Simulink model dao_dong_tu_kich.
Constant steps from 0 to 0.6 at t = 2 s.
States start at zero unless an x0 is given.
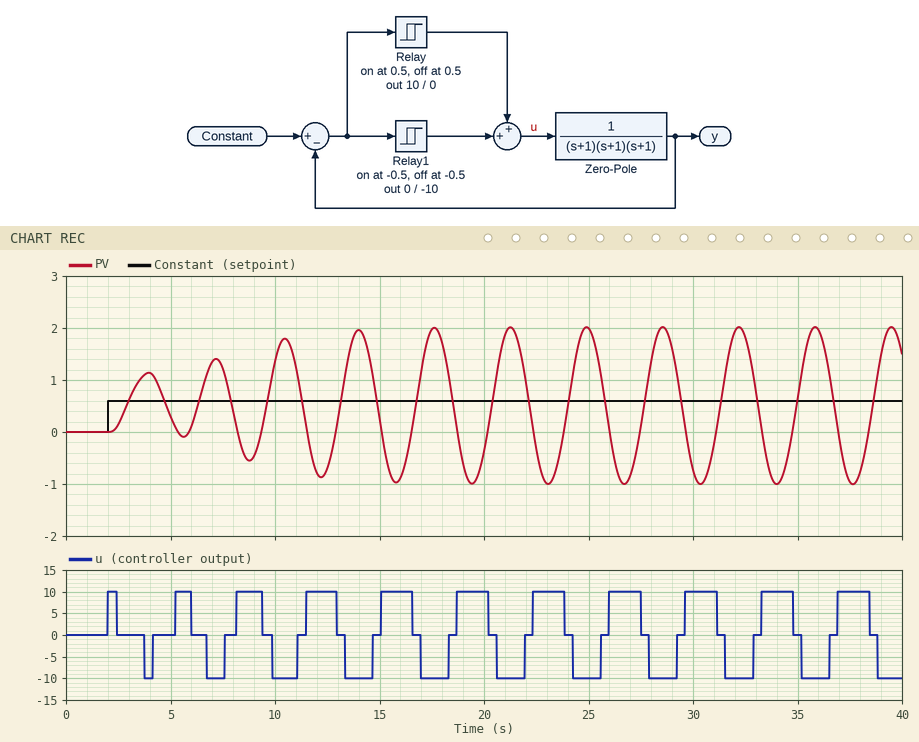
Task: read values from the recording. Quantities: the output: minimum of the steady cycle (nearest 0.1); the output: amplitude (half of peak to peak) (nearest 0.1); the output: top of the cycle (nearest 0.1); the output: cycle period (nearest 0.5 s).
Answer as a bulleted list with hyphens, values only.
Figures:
- -1.0
- 1.5
- 2.0
- 3.5 s
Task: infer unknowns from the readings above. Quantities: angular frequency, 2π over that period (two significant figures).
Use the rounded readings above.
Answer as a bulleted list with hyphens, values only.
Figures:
- 1.8 rad/s
